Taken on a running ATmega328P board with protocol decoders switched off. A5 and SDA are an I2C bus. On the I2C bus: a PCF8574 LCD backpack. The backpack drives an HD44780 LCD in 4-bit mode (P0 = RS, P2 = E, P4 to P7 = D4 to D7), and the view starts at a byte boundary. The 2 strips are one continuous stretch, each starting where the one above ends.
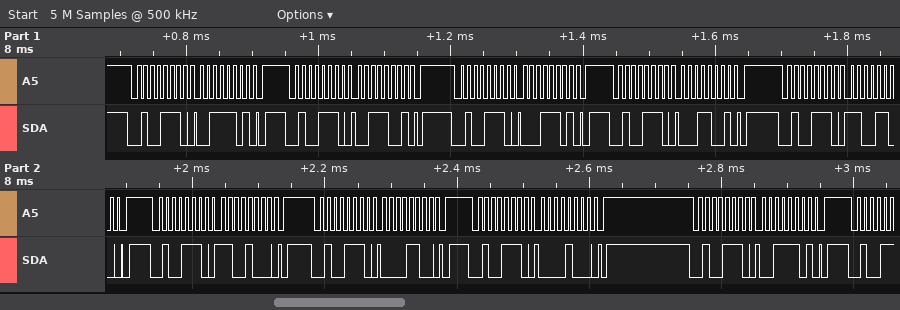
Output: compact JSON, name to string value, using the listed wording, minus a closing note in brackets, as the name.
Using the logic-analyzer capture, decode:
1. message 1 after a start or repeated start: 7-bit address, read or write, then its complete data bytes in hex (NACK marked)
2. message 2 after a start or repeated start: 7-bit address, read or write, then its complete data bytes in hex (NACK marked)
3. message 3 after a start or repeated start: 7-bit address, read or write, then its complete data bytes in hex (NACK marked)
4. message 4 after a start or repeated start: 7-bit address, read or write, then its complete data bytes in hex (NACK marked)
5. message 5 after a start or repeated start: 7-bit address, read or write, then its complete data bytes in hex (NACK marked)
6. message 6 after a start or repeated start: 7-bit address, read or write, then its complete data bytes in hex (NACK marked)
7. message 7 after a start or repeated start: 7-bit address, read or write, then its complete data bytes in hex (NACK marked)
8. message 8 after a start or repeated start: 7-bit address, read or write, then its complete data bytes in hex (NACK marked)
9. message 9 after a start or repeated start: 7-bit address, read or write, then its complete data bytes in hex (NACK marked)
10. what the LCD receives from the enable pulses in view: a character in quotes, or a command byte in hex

{"message 1 after a start or repeated start: 7-bit address, read or write, then its complete data bytes in hex": "0x27 write: 3D", "message 2 after a start or repeated start: 7-bit address, read or write, then its complete data bytes in hex": "0x27 write: 39", "message 3 after a start or repeated start: 7-bit address, read or write, then its complete data bytes in hex": "0x27 write: 1D", "message 4 after a start or repeated start: 7-bit address, read or write, then its complete data bytes in hex": "0x27 write: 19", "message 5 after a start or repeated start: 7-bit address, read or write, then its complete data bytes in hex": "0x27 write: CC", "message 6 after a start or repeated start: 7-bit address, read or write, then its complete data bytes in hex": "0x27 write: C8", "message 7 after a start or repeated start: 7-bit address, read or write, then its complete data bytes in hex": "0x27 write: 0C", "message 8 after a start or repeated start: 7-bit address, read or write, then its complete data bytes in hex": "0x27 write: 08", "message 9 after a start or repeated start: 7-bit address, read or write, then its complete data bytes in hex": "0x27 write: 3D", "what the LCD receives from the enable pulses in view: a character in quotes, or a command byte in hex": "'1' 0xC0"}
